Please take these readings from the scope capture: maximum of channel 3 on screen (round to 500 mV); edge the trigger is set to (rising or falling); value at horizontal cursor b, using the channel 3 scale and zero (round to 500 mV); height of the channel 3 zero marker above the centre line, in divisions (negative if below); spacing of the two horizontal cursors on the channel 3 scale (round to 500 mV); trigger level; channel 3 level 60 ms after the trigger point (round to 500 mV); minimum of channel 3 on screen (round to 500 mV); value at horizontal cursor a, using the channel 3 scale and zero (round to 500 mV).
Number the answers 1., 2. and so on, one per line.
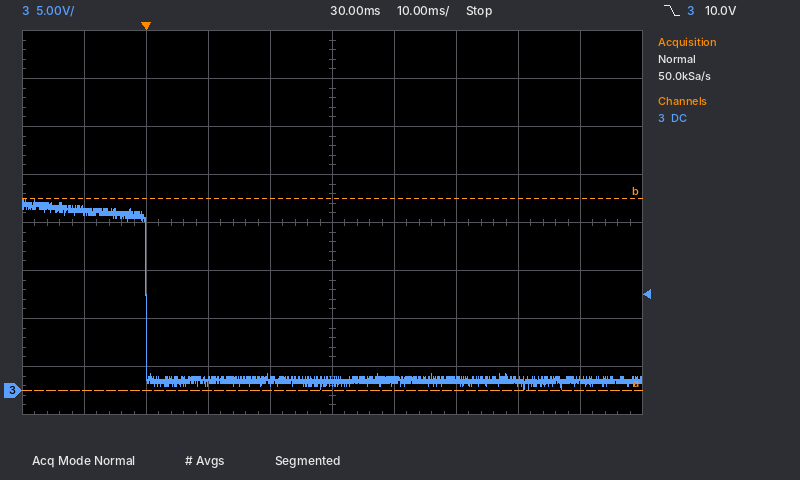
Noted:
1. 20.0 V
2. falling
3. 20.0 V
4. -3.5 div
5. 20.0 V
6. 10.0 V
7. 1.0 V
8. 0.0 V
9. 0.0 V
